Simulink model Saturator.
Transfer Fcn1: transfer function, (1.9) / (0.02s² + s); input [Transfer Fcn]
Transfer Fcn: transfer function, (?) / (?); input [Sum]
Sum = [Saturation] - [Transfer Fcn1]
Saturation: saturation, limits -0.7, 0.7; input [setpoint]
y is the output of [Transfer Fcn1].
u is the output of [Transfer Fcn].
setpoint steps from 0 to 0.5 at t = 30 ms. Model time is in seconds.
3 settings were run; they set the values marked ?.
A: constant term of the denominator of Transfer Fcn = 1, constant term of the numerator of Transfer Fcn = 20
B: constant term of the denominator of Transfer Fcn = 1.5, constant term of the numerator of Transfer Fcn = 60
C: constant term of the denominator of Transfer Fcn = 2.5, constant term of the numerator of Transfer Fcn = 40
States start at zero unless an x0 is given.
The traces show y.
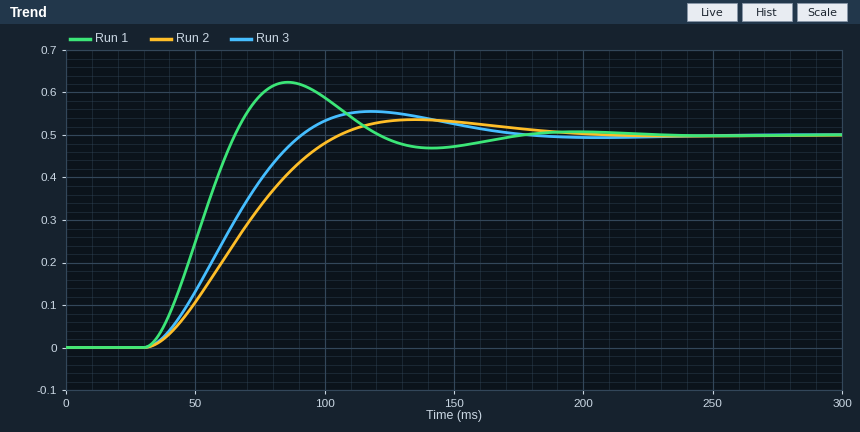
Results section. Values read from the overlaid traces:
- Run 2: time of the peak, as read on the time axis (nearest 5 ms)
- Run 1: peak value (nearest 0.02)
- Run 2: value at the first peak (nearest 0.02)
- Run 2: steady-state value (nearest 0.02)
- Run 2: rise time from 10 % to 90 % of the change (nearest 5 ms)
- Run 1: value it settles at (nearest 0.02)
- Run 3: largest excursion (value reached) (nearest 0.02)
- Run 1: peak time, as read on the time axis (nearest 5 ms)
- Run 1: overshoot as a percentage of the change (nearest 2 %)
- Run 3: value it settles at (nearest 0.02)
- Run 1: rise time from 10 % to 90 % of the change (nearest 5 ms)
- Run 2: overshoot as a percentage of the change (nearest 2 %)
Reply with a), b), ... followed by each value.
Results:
a) 135 ms
b) 0.62
c) 0.54
d) 0.50
e) 50 ms
f) 0.50
g) 0.56
h) 85 ms
i) 24 %
j) 0.50
k) 25 ms
l) 8 %
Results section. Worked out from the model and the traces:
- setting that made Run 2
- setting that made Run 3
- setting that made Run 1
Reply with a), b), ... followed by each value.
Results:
a) C
b) A
c) B
